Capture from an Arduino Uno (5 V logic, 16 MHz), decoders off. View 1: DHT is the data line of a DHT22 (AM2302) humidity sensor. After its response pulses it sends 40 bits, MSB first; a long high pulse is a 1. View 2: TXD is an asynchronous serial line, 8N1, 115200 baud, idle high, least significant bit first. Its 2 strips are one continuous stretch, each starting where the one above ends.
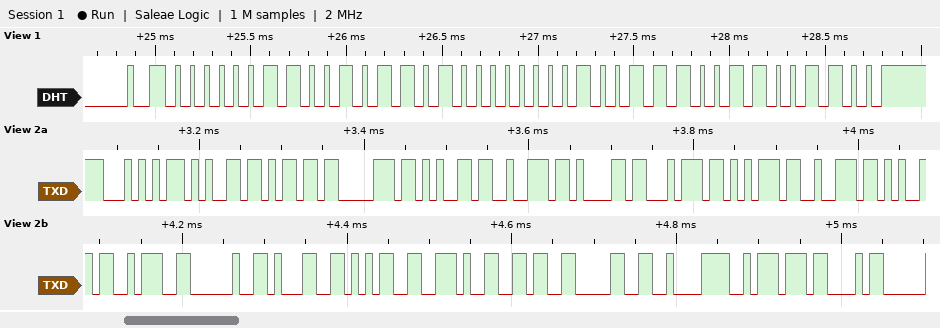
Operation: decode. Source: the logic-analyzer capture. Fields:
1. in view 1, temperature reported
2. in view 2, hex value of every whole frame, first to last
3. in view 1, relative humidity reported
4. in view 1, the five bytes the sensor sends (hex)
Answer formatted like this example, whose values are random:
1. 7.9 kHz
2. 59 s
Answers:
1. 15.6 °C
2. 54 65 6D 70 65 72 61 74 75 72 65 3A 20 31 35 2E 36 30 C2 BA 43
3. 81.3 %
4. 03 2D 00 9C CC
